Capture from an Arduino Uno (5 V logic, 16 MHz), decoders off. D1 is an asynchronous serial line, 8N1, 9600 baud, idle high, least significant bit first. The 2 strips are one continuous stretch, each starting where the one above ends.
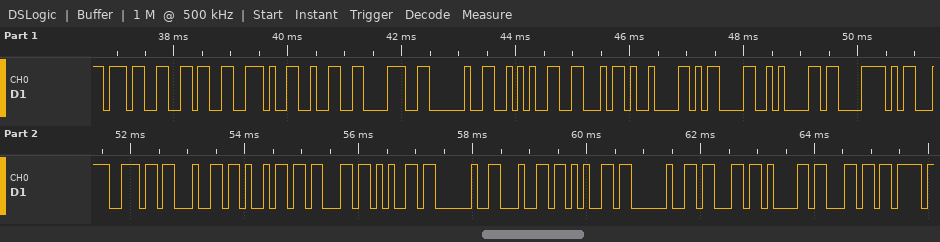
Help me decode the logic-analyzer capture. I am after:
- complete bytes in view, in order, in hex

37 36 2E 32 38 20 2A 46 09 0D 0A C3 8D 6E 64 69 63 65 20 64 65 20 63 61 6C
